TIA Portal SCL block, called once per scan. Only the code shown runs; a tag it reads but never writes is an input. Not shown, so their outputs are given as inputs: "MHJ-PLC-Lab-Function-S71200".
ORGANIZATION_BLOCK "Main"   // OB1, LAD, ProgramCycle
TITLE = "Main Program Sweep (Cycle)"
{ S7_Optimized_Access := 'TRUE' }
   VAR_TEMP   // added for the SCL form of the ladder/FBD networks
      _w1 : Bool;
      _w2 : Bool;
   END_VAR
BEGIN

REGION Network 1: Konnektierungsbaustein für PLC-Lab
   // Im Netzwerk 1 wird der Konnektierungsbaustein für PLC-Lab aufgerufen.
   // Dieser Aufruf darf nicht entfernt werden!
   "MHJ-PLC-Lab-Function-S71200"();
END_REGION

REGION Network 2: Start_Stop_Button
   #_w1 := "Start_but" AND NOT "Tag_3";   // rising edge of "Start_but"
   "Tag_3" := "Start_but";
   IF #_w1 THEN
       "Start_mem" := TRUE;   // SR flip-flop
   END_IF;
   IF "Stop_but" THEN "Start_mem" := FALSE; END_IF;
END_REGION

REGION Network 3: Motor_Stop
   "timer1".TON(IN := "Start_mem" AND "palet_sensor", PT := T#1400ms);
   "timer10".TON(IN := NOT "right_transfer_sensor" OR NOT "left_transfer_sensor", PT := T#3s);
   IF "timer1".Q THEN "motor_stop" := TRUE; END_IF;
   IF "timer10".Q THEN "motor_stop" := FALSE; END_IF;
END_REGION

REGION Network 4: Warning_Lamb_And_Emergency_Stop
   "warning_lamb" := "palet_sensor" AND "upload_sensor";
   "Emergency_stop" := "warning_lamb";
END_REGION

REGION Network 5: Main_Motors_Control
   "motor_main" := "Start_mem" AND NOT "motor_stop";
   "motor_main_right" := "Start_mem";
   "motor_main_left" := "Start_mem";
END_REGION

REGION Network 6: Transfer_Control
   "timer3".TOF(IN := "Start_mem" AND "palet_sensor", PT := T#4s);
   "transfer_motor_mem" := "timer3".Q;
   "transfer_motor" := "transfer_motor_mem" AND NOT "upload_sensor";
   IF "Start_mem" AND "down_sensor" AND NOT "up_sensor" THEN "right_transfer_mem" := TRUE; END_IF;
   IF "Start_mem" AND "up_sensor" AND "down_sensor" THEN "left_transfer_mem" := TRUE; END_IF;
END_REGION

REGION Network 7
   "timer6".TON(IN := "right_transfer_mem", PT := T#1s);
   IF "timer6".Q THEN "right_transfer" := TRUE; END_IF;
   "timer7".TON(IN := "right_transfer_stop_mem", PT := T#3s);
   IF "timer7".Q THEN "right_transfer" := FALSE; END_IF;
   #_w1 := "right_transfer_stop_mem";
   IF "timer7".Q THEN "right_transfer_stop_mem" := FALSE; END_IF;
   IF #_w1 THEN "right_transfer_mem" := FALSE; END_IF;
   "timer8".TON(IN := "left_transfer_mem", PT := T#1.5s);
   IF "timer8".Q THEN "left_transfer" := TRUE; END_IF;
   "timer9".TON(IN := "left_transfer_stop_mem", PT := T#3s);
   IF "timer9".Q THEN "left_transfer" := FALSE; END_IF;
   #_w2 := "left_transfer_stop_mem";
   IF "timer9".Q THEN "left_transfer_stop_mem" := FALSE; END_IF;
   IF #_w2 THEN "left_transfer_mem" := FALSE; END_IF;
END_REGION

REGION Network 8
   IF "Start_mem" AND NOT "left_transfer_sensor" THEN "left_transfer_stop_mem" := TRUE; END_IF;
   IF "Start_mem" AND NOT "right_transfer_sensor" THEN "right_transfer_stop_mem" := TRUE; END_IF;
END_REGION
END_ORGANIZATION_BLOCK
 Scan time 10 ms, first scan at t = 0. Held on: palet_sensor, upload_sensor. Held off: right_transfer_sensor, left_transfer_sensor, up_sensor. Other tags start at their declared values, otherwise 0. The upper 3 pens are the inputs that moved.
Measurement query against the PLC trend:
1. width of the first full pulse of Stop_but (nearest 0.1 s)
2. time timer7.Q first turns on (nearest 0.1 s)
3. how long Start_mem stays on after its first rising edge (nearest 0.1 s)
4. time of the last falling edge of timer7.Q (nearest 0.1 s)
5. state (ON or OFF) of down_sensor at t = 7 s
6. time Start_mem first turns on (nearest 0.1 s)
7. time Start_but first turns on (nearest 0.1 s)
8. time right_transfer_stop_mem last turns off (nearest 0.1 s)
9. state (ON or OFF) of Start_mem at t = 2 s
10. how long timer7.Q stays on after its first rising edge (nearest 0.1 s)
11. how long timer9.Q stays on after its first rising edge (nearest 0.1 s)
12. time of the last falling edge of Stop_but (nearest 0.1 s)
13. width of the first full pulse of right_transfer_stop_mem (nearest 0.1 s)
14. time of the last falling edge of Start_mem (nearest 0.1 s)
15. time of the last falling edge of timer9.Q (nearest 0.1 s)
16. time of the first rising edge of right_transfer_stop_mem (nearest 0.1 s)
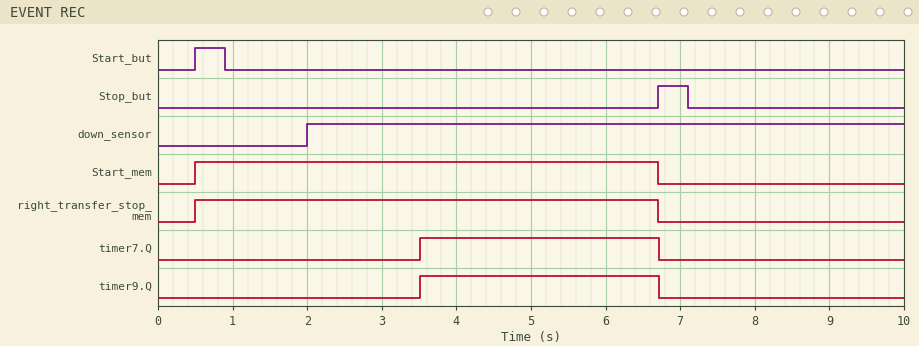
0.4 s
3.5 s
6.2 s
6.7 s
ON
0.5 s
0.5 s
6.7 s
ON
3.2 s
3.2 s
7.1 s
6.2 s
6.7 s
6.7 s
0.5 s
